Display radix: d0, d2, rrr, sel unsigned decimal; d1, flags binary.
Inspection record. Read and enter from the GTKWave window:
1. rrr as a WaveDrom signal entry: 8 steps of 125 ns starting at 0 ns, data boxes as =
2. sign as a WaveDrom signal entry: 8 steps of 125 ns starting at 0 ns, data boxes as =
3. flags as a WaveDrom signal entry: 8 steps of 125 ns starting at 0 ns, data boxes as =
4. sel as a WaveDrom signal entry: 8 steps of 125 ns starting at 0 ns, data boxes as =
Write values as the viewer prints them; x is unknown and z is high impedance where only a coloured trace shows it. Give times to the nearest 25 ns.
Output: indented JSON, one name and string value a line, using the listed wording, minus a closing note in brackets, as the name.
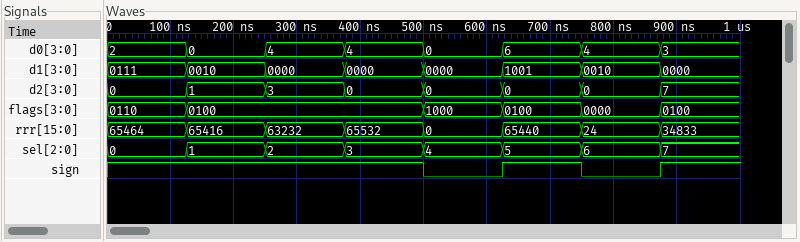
{
  "rrr as a WaveDrom signal entry: 8 steps of 125 ns starting at 0 ns, data boxes as =": "{name: 'rrr', wave: '========', data: '65464 65416 63232 65532 0 65440 24 34833'}",
  "sign as a WaveDrom signal entry: 8 steps of 125 ns starting at 0 ns, data boxes as =": "{name: 'sign', wave: '1...0101'}",
  "flags as a WaveDrom signal entry: 8 steps of 125 ns starting at 0 ns, data boxes as =": "{name: 'flags', wave: '==..====', data: '0110 0100 1000 0100 0000 0100'}",
  "sel as a WaveDrom signal entry: 8 steps of 125 ns starting at 0 ns, data boxes as =": "{name: 'sel', wave: '========', data: '0 1 2 3 4 5 6 7'}"
}
